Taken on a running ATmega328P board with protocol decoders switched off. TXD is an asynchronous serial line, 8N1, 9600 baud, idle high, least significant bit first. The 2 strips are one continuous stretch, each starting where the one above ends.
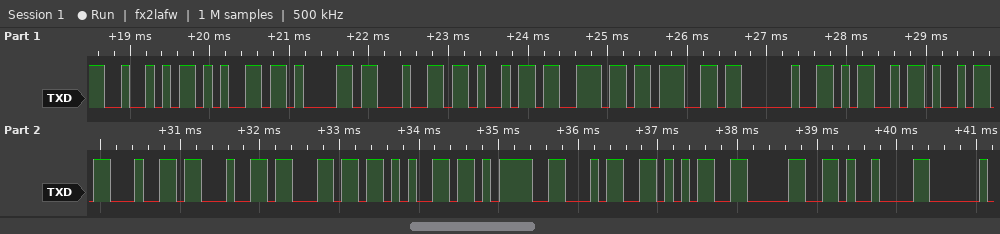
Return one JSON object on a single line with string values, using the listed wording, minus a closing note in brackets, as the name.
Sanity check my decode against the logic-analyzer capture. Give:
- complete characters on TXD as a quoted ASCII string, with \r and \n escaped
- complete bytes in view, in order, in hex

{"complete characters on TXD as a quoted ASCII string, with \\r and \\n escaped": "\"Reading Middle=450\\t\"", "complete bytes in view, in order, in hex": "0x52 0x65 0x61 0x64 0x69 0x6E 0x67 0x20 0x4D 0x69 0x64 0x64 0x6C 0x65 0x3D 0x34 0x35 0x30 0x09"}
